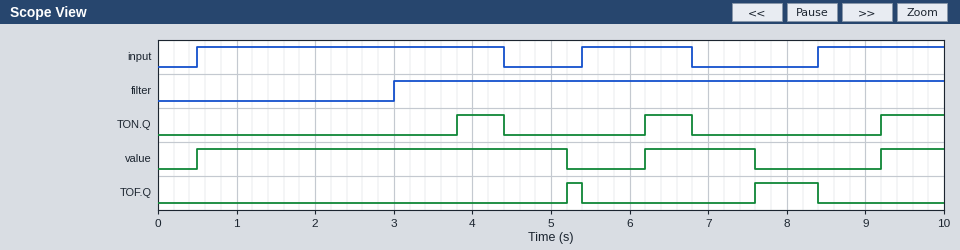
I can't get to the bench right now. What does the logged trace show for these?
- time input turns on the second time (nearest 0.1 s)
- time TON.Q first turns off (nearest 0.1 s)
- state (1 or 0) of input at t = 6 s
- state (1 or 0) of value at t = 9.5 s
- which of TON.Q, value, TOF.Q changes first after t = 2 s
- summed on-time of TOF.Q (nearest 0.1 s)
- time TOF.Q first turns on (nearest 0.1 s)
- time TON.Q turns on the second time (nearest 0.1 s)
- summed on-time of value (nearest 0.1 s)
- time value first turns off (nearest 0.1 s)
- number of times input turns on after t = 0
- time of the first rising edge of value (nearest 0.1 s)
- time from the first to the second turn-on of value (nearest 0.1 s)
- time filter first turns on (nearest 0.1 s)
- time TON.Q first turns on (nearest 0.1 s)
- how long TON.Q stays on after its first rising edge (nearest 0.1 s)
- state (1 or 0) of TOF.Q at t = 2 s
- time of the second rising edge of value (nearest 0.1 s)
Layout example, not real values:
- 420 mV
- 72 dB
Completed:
- 5.4 s
- 4.4 s
- 1
- 1
- TON.Q
- 1.0 s
- 5.2 s
- 6.2 s
- 6.9 s
- 5.2 s
- 3
- 0.5 s
- 5.7 s
- 3.0 s
- 3.8 s
- 0.6 s
- 0
- 6.2 s
